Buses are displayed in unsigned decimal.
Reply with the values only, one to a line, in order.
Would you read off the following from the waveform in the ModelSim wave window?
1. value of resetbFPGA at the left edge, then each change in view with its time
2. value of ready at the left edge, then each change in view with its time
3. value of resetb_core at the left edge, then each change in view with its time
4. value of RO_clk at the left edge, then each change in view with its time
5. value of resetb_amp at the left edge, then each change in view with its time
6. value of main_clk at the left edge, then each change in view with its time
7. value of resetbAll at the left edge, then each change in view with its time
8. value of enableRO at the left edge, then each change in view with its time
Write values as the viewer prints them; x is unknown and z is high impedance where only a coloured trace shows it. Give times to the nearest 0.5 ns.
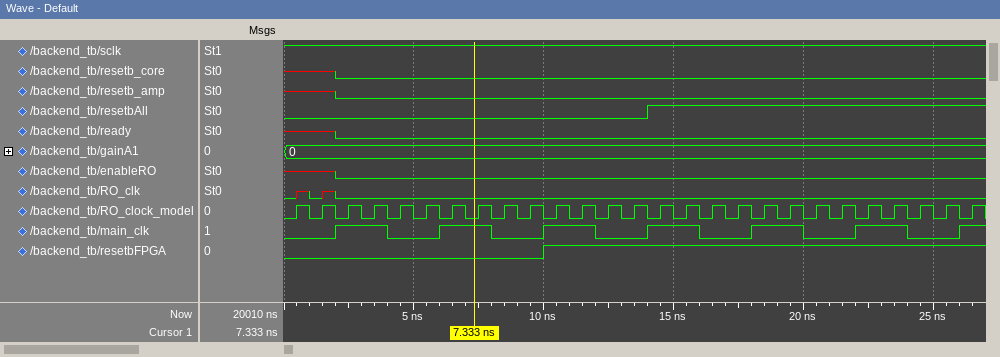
0, 1 at 10 ns
x, 0 at 2 ns
x, 0 at 2 ns
0, x at 0.5 ns, 0 at 1 ns, x at 1.5 ns, 0 at 2 ns
x, 0 at 2 ns
0, 1 at 2 ns, 0 at 4 ns, 1 at 6 ns, 0 at 8 ns, 1 at 10 ns, 0 at 12 ns, 1 at 14 ns, 0 at 16 ns, 1 at 18 ns, 0 at 20 ns, 1 at 22 ns, 0 at 24 ns, 1 at 26 ns
0, 1 at 14 ns
x, 0 at 2 ns
